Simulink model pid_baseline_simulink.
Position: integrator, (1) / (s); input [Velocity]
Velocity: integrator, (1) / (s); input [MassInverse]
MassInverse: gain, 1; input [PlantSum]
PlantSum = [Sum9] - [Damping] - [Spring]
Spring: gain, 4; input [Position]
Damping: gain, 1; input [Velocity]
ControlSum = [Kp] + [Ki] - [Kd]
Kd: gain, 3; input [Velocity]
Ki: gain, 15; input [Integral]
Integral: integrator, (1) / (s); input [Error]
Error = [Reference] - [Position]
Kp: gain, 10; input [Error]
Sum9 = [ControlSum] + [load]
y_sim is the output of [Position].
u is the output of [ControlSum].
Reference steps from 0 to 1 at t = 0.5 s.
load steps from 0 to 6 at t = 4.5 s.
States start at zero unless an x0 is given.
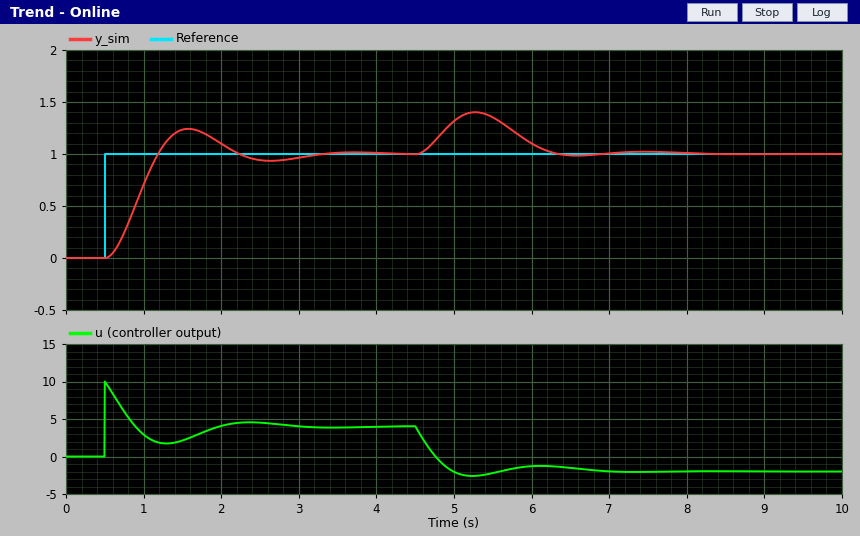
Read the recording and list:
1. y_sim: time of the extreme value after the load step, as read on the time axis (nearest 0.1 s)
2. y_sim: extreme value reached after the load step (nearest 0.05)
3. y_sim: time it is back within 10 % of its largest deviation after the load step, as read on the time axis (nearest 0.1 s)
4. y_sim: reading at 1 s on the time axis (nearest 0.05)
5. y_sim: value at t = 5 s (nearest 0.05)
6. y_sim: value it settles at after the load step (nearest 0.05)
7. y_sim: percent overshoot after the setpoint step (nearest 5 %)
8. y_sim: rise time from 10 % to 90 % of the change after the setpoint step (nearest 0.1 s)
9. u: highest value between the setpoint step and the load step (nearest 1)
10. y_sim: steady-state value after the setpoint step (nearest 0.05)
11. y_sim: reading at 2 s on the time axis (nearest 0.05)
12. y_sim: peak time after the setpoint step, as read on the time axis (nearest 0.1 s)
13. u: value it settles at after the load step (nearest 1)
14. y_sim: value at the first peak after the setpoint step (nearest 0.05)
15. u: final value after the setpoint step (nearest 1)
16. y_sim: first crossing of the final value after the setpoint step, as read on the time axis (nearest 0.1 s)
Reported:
5.3 s
1.40
6.2 s
0.70
1.30
1.00
25 %
0.5 s
10
1.00
1.10
1.6 s
-2
1.25
4
1.2 s
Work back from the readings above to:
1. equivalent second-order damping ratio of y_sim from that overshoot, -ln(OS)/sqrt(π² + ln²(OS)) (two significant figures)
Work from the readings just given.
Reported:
0.40
